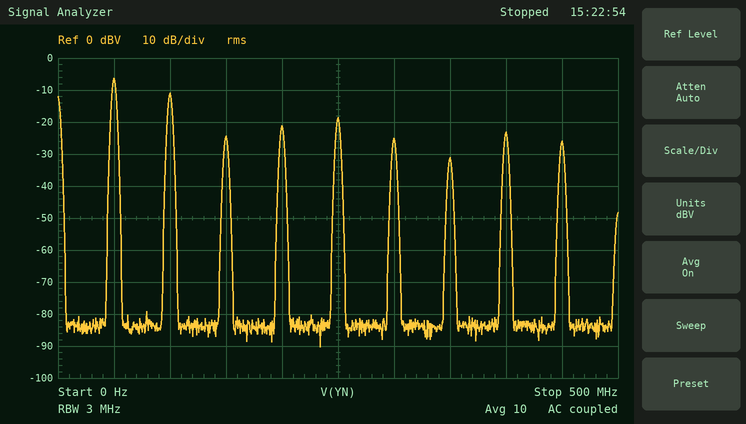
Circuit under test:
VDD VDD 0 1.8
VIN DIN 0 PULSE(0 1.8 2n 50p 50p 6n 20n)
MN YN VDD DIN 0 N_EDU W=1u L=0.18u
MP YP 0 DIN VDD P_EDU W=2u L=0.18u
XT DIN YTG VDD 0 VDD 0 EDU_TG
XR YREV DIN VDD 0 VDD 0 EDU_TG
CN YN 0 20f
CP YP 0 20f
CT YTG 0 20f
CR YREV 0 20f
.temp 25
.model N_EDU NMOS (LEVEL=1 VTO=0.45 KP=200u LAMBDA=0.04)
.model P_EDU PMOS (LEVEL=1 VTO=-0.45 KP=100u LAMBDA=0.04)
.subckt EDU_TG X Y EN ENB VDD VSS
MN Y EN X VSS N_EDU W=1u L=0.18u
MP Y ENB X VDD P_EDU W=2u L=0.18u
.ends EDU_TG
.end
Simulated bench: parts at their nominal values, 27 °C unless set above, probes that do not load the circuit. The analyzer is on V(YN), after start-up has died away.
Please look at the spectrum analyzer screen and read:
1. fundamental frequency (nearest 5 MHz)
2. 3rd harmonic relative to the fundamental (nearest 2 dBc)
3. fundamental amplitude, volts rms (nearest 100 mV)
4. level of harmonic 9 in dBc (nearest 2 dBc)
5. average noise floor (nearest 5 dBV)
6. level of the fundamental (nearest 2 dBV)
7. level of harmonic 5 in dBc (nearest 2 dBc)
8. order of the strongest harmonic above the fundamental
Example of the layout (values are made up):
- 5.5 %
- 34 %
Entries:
- 50 MHz
- -18 dBc
- 500 mV
- -20 dBc
- -85 dBV
- -6 dBV
- -12 dBc
- 2
